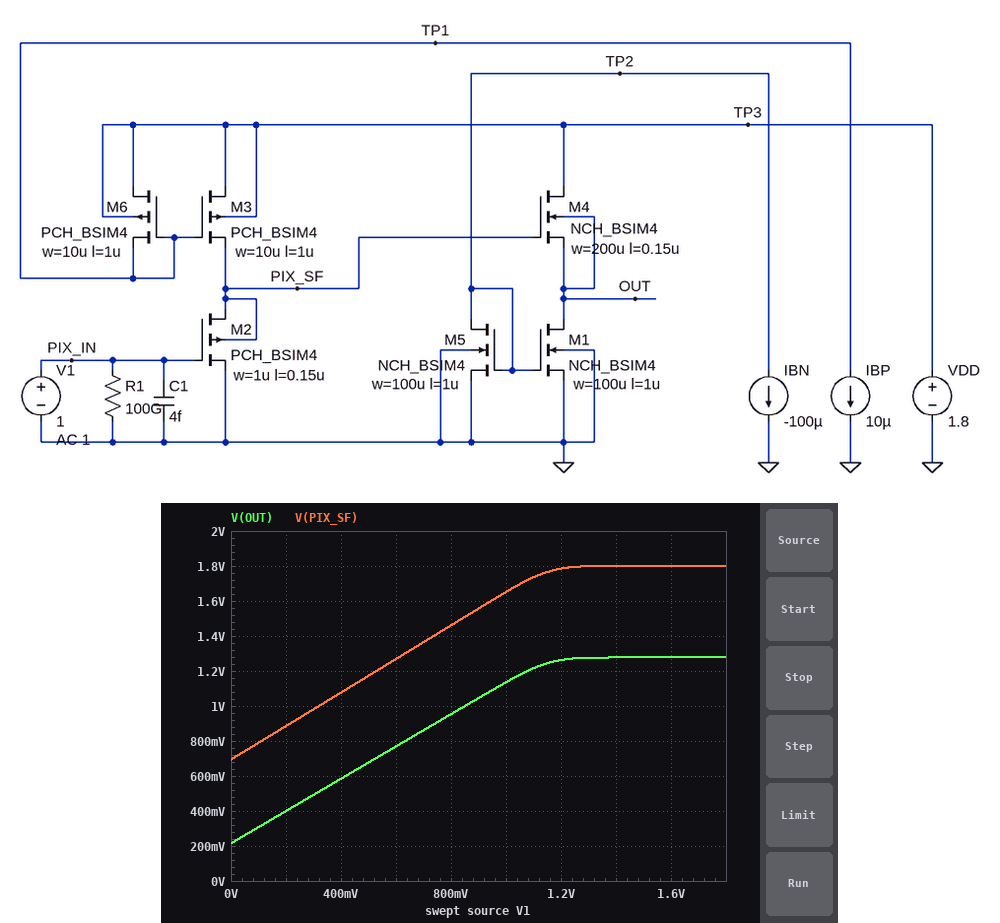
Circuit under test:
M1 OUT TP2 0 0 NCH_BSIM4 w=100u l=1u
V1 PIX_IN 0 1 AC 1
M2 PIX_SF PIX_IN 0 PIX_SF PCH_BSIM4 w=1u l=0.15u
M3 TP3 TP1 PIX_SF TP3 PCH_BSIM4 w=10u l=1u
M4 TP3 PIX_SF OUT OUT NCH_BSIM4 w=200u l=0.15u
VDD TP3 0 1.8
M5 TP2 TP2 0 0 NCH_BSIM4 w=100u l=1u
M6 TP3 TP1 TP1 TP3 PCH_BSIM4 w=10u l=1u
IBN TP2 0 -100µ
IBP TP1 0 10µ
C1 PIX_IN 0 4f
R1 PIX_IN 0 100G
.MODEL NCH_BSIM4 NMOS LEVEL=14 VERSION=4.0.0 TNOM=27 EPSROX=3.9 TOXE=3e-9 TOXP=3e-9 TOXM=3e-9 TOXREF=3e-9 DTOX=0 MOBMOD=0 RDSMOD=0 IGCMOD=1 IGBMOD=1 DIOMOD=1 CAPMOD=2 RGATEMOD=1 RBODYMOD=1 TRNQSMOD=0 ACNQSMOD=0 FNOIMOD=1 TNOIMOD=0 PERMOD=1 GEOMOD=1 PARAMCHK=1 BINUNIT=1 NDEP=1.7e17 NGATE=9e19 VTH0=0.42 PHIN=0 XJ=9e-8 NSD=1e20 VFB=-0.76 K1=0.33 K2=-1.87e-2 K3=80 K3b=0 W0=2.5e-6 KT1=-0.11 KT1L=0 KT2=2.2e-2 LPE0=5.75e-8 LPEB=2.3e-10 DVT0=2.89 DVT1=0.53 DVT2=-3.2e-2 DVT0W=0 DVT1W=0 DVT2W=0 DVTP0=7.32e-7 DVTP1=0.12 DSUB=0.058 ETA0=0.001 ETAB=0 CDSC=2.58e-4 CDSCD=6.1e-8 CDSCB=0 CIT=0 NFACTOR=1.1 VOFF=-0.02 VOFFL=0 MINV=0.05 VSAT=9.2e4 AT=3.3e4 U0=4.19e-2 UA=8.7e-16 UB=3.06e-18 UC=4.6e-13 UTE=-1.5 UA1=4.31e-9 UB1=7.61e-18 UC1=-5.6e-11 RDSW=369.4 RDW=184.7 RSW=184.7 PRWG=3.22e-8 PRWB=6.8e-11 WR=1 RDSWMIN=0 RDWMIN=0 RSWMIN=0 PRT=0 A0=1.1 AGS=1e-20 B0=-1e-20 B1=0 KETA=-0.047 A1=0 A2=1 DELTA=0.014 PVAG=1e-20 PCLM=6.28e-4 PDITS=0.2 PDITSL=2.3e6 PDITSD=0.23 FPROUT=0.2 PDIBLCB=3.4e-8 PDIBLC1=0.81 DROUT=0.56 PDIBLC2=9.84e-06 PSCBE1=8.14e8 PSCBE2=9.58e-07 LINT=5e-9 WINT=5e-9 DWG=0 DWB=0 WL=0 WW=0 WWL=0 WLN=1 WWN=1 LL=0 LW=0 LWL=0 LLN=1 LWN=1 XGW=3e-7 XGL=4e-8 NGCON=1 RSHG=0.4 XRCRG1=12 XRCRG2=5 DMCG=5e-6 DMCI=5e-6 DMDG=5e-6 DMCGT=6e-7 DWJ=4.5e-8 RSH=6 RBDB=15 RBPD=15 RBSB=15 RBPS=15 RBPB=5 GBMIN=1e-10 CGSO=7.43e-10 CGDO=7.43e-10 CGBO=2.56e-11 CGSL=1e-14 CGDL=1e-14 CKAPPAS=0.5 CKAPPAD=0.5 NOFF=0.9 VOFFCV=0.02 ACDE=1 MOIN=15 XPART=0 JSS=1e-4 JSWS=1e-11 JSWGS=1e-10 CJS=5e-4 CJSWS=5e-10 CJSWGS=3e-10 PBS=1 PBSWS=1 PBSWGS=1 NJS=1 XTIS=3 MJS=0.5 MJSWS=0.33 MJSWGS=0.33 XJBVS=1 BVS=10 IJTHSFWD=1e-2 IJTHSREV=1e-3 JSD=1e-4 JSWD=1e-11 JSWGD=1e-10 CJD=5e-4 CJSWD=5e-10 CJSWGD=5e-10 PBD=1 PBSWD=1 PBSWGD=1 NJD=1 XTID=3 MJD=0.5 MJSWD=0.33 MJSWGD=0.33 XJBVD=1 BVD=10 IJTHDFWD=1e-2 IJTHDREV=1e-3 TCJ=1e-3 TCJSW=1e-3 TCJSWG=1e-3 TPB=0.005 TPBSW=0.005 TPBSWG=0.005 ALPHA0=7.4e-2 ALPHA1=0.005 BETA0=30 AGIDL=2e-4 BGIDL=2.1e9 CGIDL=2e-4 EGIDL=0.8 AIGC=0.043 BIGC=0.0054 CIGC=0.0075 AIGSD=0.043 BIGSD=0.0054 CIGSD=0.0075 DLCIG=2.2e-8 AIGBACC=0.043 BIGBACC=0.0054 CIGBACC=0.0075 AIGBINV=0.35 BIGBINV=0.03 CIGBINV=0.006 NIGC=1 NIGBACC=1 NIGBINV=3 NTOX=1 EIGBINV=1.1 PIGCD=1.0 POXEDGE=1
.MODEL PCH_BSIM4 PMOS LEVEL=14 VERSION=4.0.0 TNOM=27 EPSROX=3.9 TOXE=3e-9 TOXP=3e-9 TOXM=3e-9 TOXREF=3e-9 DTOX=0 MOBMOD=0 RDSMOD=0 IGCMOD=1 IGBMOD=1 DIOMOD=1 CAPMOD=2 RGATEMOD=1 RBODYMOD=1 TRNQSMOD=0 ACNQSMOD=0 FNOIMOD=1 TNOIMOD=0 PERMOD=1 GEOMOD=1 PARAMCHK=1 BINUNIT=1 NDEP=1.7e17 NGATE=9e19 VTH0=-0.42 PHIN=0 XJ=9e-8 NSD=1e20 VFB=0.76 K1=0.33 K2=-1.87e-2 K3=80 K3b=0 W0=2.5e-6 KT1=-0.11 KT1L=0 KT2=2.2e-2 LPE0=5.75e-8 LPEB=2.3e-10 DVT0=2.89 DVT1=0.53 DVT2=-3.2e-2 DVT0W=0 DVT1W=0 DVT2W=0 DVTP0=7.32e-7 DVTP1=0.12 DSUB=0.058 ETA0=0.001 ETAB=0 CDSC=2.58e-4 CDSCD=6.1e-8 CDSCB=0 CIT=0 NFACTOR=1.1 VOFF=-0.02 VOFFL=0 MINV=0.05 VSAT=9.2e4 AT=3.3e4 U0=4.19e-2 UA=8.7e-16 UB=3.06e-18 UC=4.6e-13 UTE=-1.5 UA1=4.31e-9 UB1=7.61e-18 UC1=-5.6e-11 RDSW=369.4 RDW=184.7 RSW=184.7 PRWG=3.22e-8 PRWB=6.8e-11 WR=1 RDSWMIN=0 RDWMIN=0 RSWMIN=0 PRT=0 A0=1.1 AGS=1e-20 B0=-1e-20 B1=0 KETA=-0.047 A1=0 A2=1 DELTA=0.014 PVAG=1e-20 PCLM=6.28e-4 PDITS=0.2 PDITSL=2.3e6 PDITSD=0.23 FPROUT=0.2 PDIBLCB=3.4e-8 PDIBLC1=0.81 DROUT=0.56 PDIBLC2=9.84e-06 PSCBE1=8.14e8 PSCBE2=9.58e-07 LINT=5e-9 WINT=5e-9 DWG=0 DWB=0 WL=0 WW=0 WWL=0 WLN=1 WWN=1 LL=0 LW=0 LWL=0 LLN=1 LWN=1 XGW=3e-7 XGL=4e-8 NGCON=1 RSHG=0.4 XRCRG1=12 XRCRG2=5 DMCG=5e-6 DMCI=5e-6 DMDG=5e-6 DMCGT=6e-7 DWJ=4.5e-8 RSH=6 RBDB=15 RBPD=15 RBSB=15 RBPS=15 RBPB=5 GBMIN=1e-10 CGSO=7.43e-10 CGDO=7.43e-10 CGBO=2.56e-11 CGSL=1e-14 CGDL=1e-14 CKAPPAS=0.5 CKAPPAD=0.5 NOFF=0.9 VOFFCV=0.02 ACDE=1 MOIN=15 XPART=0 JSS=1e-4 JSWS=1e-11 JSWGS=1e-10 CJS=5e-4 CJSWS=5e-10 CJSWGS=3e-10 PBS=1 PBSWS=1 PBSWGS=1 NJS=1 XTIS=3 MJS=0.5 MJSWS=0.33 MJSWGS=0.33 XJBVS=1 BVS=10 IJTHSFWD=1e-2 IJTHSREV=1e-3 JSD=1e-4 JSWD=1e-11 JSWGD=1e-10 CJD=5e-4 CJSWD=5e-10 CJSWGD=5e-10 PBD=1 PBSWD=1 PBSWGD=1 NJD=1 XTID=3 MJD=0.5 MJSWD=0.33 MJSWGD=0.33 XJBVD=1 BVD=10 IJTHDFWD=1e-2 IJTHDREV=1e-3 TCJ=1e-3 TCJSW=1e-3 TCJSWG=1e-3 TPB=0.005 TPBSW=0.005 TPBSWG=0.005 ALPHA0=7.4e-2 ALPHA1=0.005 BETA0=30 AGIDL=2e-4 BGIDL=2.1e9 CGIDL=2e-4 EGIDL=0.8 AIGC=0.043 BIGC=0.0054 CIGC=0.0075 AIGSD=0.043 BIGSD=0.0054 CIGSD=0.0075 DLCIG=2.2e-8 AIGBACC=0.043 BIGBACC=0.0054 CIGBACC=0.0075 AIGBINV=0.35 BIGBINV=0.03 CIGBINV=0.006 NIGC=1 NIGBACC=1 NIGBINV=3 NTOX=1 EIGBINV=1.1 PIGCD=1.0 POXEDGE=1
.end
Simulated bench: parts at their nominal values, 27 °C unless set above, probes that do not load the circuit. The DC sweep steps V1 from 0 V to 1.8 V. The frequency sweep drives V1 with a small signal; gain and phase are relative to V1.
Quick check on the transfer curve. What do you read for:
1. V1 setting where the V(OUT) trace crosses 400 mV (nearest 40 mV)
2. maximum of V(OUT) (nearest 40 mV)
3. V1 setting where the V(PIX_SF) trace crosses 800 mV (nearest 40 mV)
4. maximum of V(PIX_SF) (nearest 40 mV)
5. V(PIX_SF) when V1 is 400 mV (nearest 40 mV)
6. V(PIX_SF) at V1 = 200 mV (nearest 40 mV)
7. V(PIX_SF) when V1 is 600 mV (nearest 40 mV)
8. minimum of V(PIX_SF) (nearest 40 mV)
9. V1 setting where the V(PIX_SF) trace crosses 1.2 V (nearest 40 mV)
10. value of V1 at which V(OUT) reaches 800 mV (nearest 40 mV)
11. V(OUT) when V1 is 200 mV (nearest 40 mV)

200 mV
1.28 V
120 mV
1.80 V
1.08 V
880 mV
1.28 V
680 mV
520 mV
640 mV
400 mV
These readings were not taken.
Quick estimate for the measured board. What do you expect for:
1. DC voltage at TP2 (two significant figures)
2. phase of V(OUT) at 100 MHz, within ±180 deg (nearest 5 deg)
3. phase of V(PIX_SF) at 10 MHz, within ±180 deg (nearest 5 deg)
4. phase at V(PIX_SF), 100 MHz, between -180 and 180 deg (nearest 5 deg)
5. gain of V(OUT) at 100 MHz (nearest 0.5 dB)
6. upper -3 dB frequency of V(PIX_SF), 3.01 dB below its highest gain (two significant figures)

590 mV
-55 deg
-5 deg
-45 deg
-3.5 dB
120 MHz
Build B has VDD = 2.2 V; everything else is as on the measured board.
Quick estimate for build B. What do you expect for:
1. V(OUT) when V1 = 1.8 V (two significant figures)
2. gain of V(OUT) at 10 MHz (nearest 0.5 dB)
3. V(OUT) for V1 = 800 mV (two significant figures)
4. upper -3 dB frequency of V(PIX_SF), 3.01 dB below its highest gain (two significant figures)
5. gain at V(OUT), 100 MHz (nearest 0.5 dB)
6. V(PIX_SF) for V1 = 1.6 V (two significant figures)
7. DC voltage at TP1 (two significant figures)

1.7 V
-0.5 dB
970 mV
130 MHz
-3.0 dB
2.2 V
1.6 V
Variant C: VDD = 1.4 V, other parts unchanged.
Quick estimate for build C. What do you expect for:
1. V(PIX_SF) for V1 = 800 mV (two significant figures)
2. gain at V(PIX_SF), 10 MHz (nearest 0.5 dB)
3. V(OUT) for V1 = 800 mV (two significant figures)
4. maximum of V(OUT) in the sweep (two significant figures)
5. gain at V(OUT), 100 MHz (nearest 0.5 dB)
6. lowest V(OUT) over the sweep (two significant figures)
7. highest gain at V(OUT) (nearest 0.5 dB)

1.4 V
-58.5 dB
870 mV
880 mV
-52.0 dB
200 mV
-51.5 dB
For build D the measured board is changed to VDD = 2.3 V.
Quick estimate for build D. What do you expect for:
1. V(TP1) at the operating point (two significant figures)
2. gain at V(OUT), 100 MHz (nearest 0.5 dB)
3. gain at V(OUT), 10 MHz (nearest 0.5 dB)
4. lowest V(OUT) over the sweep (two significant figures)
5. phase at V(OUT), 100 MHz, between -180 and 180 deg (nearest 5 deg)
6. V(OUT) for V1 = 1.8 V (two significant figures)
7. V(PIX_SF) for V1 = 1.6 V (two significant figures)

1.7 V
-3.0 dB
-0.5 dB
240 mV
-50 deg
1.8 V
2.2 V
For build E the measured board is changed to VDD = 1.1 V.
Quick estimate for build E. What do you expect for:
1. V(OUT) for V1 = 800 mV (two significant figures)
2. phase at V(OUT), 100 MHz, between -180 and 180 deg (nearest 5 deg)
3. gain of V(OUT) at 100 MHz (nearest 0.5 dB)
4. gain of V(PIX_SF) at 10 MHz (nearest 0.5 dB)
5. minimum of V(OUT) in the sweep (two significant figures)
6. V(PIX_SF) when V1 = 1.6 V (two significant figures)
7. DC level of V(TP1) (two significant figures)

580 mV
25 deg
-52.0 dB
-68.0 dB
190 mV
1.1 V
500 mV
